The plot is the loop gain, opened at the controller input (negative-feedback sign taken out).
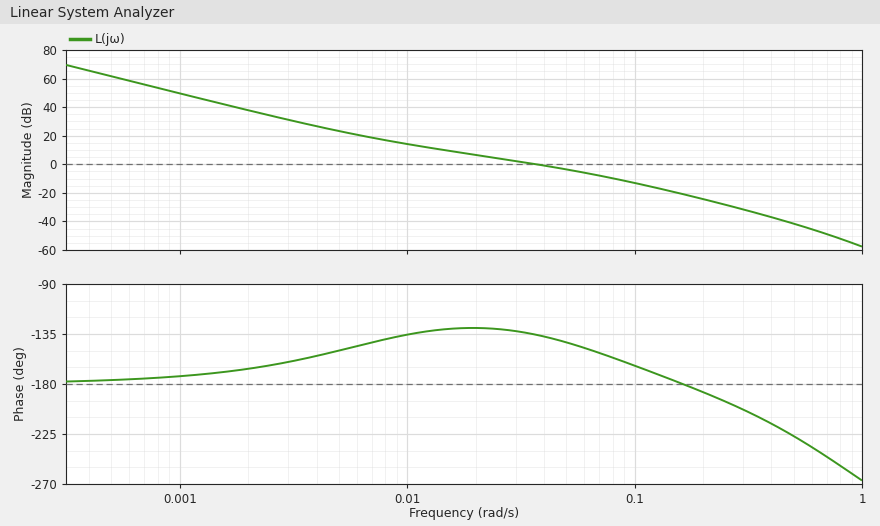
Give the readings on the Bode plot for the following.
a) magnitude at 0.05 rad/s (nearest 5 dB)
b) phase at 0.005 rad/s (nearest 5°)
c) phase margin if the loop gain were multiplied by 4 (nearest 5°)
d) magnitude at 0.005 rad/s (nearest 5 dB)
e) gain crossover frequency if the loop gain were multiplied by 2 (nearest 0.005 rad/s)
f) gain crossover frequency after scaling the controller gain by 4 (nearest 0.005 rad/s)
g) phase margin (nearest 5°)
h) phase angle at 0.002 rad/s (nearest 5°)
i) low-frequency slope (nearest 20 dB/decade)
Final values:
-5 dB
-150°
20°
25 dB
0.060 rad/s
0.095 rad/s
45°
-165°
-40 dB/decade
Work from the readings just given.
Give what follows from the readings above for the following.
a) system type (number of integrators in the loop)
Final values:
2
